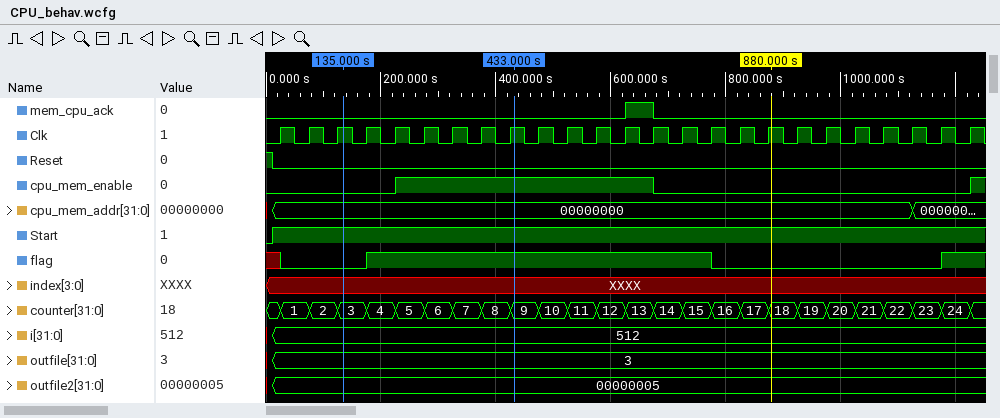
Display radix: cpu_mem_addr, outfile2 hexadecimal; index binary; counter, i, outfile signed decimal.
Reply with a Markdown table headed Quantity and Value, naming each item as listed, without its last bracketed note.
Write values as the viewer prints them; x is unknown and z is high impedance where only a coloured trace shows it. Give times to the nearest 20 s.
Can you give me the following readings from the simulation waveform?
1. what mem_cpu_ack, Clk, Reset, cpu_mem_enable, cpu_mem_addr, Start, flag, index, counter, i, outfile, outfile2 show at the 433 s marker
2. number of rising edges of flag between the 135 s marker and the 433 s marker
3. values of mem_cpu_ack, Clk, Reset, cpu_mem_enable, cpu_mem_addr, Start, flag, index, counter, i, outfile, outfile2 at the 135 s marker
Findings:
| Quantity | Value |
|---|---|
| what mem_cpu_ack, Clk, Reset, cpu_mem_enable, cpu_mem_addr, Start, flag, index, counter, i, outfile, outfile2 show at the 433 s marker | mem_cpu_ack=0, Clk=1, Reset=0, cpu_mem_enable=1, cpu_mem_addr=00000000, Start=1, flag=1, index=XXXX, counter=9, i=512, outfile=3, outfile2=00000005 |
| number of rising edges of flag between the 135 s marker and the 433 s marker | 1 |
| values of mem_cpu_ack, Clk, Reset, cpu_mem_enable, cpu_mem_addr, Start, flag, index, counter, i, outfile, outfile2 at the 135 s marker | mem_cpu_ack=0, Clk=1, Reset=0, cpu_mem_enable=0, cpu_mem_addr=00000000, Start=1, flag=0, index=XXXX, counter=3, i=512, outfile=3, outfile2=00000005 |
